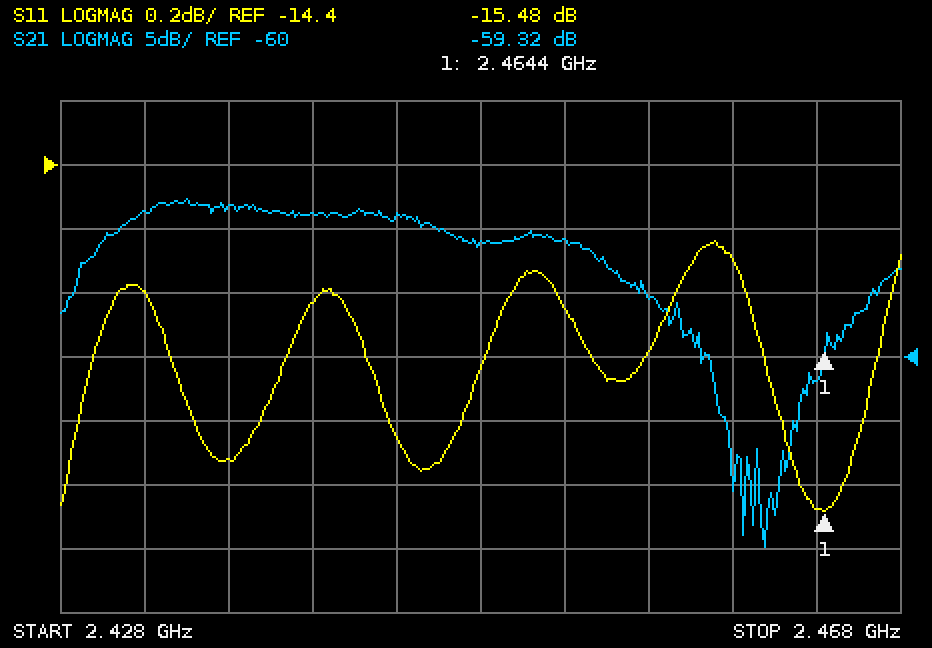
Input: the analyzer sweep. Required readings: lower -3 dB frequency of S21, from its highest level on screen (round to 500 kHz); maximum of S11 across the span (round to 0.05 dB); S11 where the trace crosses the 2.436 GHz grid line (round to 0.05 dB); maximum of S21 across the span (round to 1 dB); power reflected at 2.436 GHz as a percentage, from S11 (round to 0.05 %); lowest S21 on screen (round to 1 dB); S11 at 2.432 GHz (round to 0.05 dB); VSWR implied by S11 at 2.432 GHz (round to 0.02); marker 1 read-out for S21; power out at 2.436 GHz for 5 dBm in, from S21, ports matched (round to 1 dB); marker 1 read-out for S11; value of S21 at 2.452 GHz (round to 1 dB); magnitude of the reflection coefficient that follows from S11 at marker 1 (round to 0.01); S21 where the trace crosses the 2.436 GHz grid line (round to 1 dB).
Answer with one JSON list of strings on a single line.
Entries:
["2.4300 GHz", "-14.65 dB", "-15.30 dB", "-48 dB", "2.95 %", "-75 dB", "-14.80 dB", "1.44", "-59.32 dB", "-43 dBm", "-15.48 dB", "-51 dB", "0.17", "-48 dB"]
